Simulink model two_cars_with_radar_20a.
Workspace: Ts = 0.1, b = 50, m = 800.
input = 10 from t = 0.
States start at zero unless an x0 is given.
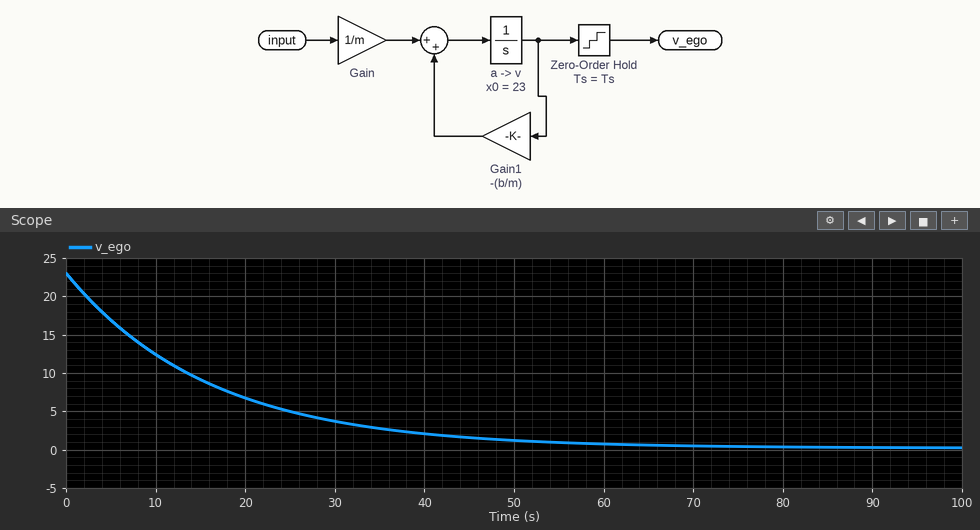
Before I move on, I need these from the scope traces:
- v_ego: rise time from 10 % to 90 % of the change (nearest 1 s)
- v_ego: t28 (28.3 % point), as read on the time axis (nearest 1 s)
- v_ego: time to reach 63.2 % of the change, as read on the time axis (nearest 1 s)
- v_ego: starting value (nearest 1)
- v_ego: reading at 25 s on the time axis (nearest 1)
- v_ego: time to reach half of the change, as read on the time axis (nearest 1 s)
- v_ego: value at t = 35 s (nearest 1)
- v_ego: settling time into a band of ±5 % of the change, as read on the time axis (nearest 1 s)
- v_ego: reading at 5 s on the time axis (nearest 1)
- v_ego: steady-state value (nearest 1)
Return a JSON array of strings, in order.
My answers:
["35 s", "5 s", "16 s", "23", "5", "11 s", "3", "48 s", "17", "0"]
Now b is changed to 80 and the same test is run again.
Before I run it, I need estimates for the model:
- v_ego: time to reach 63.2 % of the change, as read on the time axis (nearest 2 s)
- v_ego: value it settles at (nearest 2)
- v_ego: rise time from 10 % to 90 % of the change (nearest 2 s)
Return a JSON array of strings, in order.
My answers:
["10 s", "0", "22 s"]
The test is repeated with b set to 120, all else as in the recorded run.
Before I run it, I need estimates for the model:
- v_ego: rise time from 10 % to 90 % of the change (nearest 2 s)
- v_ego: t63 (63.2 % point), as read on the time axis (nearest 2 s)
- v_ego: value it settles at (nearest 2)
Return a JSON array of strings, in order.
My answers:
["14 s", "6 s", "0"]
